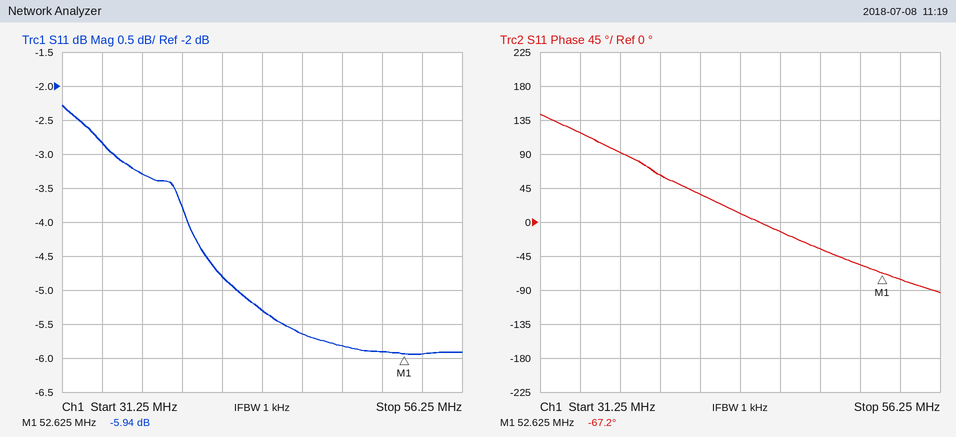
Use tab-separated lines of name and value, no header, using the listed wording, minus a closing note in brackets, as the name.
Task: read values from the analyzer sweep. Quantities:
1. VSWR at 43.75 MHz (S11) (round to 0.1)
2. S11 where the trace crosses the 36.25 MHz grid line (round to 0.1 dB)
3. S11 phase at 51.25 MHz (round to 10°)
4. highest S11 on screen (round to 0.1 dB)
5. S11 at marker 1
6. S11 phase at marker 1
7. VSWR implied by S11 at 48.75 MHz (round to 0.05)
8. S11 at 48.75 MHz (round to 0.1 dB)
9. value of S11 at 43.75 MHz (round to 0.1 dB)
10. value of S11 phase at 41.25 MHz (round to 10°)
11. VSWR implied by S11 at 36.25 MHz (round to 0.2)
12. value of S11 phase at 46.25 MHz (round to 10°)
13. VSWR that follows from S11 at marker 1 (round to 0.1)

VSWR at 43.75 MHz (S11)	3.4
S11 where the trace crosses the 36.25 MHz grid line	-3.3 dB
S11 phase at 51.25 MHz	-60°
highest S11 on screen	-2.3 dB
S11 at marker 1	-5.94 dB
S11 phase at marker 1	-67.2°
VSWR implied by S11 at 48.75 MHz	3.10
S11 at 48.75 MHz	-5.8 dB
value of S11 at 43.75 MHz	-5.3 dB
value of S11 phase at 41.25 MHz	40°
VSWR implied by S11 at 36.25 MHz	5.4
value of S11 phase at 46.25 MHz	-10°
VSWR that follows from S11 at marker 1	3.0
